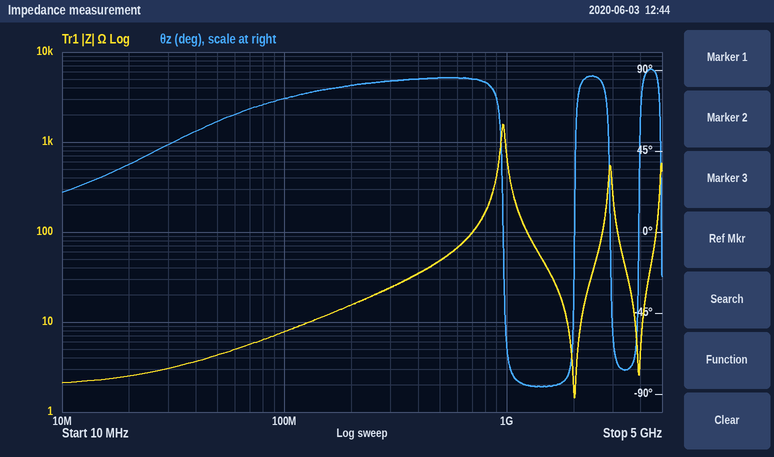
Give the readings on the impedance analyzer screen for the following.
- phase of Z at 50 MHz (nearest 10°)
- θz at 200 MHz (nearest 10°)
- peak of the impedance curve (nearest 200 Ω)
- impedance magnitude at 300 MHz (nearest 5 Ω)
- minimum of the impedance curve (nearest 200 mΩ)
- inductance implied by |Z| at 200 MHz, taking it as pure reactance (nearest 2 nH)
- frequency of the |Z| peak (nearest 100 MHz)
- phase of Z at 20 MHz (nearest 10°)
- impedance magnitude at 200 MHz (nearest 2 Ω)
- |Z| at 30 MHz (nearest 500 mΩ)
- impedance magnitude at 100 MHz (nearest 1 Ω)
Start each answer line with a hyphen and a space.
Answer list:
- 60°
- 80°
- 1.6 kΩ
- 25 Ω
- 1.4 Ω
- 12 nH
- 1.0 GHz
- 40°
- 16 Ω
- 3.0 Ω
- 8 Ω
